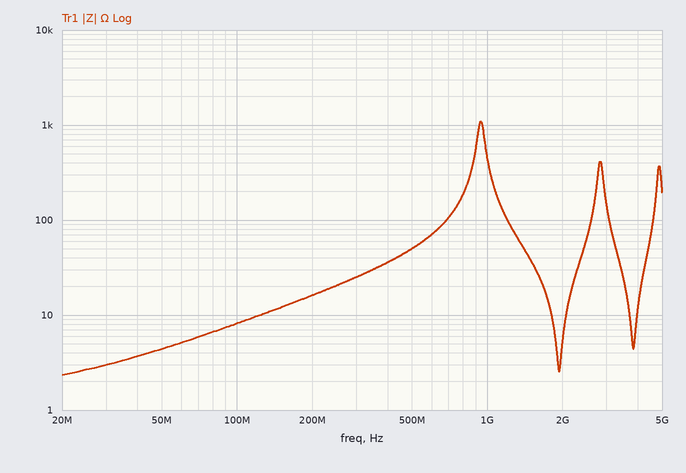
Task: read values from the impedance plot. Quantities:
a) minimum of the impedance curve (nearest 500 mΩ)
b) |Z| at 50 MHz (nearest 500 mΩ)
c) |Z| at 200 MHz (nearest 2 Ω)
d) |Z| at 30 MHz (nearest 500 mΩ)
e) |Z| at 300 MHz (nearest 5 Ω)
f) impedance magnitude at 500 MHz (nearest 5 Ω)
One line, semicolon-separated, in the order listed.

2.5 Ω; 4.5 Ω; 16 Ω; 3.0 Ω; 25 Ω; 50 Ω
